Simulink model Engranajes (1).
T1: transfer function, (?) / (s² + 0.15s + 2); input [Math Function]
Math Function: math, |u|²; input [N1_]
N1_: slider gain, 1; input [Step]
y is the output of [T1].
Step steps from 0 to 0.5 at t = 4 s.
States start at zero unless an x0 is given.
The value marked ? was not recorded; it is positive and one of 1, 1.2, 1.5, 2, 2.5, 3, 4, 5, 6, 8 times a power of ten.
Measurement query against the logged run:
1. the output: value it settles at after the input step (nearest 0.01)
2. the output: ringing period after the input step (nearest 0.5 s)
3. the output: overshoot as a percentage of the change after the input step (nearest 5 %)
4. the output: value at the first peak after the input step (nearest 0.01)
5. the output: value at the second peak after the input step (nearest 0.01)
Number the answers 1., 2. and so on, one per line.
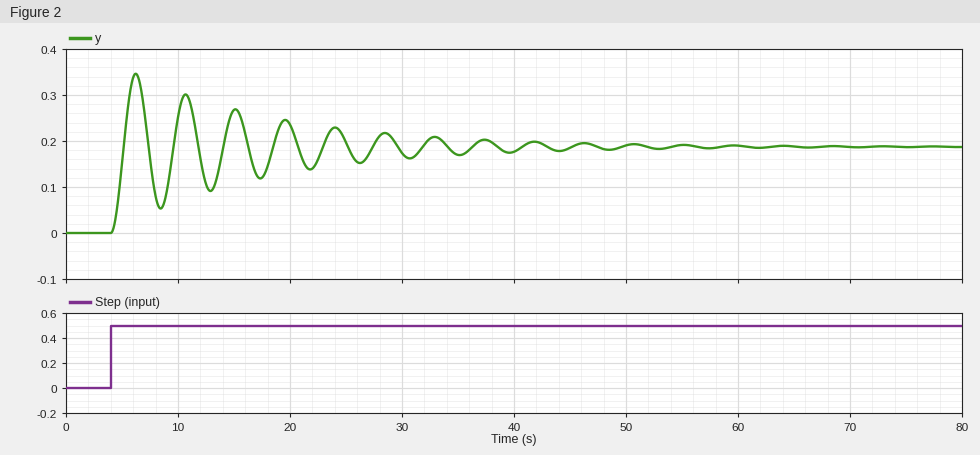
1. 0.19
2. 4.5 s
3. 85 %
4. 0.35
5. 0.30
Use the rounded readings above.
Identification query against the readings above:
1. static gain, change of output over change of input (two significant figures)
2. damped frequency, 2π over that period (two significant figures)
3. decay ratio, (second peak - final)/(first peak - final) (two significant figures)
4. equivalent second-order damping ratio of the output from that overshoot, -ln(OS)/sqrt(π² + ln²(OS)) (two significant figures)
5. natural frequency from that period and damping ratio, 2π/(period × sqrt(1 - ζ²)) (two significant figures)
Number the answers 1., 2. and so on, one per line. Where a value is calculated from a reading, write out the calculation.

1. (0.19 - 0) / (0.5 - 0) = 0.38
2. 2π / 4.5 = 1.4 rad/s
3. (0.3 - 0.19) / (0.35 - 0.19) = 0.69
4. ln(0.85) = -0.163; 0.163 / sqrt(9.870 + 0.026) = 0.052
5. 2π / (4.5 × sqrt(1 - 0.052²)) = 1.4 rad/s
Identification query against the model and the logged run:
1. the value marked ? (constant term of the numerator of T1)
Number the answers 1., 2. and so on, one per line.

1. 1.5
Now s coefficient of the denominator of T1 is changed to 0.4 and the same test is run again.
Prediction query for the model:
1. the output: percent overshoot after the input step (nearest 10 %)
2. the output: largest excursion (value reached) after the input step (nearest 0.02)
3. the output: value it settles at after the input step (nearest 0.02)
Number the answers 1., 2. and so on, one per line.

1. 60 %
2. 0.30
3. 0.18
